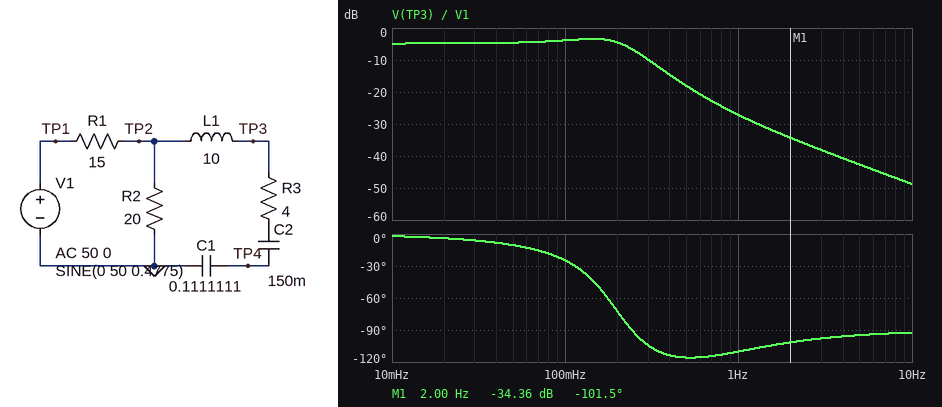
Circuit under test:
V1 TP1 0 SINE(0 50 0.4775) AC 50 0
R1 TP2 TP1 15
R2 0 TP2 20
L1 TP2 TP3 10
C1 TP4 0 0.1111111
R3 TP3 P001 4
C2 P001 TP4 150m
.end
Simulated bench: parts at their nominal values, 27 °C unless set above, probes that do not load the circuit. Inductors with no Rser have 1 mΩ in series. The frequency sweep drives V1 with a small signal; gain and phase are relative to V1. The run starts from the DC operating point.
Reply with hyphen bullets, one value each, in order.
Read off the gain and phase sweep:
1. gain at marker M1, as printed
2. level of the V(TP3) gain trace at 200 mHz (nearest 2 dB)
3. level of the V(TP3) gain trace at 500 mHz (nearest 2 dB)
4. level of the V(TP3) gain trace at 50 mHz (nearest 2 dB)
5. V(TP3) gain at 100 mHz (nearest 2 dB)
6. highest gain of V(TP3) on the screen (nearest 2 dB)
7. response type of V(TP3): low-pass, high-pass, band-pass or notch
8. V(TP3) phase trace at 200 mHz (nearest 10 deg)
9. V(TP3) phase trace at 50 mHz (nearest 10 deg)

- -34.36 dB
- -4 dB
- -18 dB
- -4 dB
- -4 dB
- -4 dB
- low-pass
- -70 deg
- -10 deg
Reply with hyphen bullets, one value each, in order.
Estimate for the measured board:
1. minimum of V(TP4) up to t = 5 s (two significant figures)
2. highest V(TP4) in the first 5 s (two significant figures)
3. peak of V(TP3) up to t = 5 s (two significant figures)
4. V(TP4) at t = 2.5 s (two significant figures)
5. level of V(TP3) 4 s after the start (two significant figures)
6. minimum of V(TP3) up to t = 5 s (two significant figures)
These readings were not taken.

- -3.5 V
- 6.7 V
- 13 V
- -2.6 V
- -4.6 V
- -7.5 V
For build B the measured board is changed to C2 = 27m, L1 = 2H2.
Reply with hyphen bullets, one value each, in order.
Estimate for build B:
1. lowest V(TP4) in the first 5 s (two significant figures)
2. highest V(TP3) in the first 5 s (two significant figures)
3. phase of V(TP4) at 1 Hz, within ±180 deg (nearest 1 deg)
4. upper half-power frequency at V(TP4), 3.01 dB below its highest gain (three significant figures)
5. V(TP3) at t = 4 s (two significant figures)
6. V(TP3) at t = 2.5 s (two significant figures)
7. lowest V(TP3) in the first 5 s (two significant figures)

- -5.6 V
- 30 V
- -117 deg
- 796 mHz
- -28 V
- 14 V
- -30 V
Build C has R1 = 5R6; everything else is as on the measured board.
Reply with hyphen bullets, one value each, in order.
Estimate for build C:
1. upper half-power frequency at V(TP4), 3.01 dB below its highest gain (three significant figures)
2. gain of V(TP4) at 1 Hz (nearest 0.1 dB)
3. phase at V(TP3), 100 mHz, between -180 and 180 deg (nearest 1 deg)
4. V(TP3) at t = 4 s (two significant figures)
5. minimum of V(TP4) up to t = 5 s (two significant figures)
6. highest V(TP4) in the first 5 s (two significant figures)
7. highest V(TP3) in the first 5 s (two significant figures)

- 236 mHz
- -34.7 dB
- -15 deg
- -7.1 V
- -5.6 V
- 11 V
- 21 V
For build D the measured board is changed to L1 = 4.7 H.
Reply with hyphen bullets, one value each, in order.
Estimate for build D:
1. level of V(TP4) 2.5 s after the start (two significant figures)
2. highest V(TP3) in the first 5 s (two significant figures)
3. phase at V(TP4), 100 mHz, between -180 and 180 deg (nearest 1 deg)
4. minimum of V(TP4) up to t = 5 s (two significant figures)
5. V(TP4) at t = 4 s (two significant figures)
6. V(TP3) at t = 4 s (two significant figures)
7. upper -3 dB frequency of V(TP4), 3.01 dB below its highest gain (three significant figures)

- -4.7 V
- 16 V
- -30 deg
- -5.6 V
- -2.2 V
- -11 V
- 280 mHz
